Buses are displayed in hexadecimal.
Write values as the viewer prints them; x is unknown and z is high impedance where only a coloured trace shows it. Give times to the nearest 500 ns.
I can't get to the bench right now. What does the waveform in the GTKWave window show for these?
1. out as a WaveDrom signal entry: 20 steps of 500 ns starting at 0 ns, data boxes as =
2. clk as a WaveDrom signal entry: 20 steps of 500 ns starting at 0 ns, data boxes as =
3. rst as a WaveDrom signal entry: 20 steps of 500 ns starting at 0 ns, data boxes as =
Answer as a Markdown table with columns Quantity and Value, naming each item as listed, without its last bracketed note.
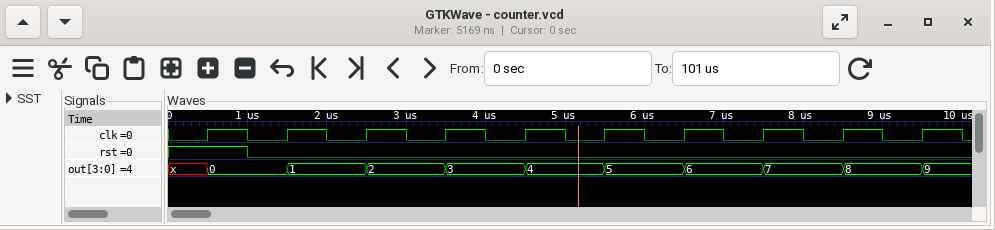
| Quantity | Value |
|---|---|
| out as a WaveDrom signal entry: 20 steps of 500 ns starting at 0 ns, data boxes as = | {name: 'out', wave: 'x=.=.=.=.=.=.=.=.=.=', data: '0 1 2 3 4 5 6 7 8 9'} |
| clk as a WaveDrom signal entry: 20 steps of 500 ns starting at 0 ns, data boxes as = | {name: 'clk', wave: '01010101010101010101'} |
| rst as a WaveDrom signal entry: 20 steps of 500 ns starting at 0 ns, data boxes as = | {name: 'rst', wave: '1.0.................'} |
